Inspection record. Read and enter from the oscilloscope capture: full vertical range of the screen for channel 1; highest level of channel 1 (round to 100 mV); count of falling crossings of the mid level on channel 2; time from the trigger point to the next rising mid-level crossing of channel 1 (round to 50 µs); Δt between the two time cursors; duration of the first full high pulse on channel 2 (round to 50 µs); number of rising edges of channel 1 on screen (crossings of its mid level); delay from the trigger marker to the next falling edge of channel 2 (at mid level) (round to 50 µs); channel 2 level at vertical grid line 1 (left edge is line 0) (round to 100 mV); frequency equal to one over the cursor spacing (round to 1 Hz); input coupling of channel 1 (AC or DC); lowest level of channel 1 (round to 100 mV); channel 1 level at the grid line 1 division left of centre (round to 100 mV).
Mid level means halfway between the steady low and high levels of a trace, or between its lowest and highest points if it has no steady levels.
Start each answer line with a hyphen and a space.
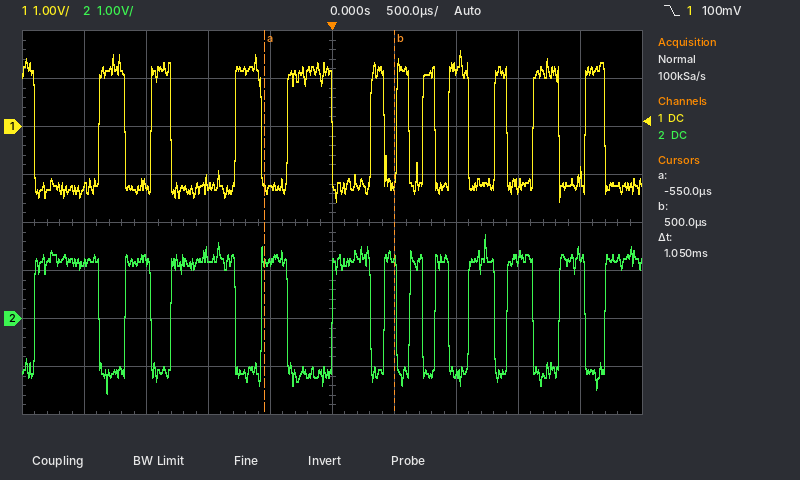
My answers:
- 8 V
- 1.6 V
- 11
- 300 µs
- 1.05 ms
- 500 µs
- 11
- 300 µs
- 1.2 V
- 952 Hz
- DC
- -1.6 V
- -1.3 V
